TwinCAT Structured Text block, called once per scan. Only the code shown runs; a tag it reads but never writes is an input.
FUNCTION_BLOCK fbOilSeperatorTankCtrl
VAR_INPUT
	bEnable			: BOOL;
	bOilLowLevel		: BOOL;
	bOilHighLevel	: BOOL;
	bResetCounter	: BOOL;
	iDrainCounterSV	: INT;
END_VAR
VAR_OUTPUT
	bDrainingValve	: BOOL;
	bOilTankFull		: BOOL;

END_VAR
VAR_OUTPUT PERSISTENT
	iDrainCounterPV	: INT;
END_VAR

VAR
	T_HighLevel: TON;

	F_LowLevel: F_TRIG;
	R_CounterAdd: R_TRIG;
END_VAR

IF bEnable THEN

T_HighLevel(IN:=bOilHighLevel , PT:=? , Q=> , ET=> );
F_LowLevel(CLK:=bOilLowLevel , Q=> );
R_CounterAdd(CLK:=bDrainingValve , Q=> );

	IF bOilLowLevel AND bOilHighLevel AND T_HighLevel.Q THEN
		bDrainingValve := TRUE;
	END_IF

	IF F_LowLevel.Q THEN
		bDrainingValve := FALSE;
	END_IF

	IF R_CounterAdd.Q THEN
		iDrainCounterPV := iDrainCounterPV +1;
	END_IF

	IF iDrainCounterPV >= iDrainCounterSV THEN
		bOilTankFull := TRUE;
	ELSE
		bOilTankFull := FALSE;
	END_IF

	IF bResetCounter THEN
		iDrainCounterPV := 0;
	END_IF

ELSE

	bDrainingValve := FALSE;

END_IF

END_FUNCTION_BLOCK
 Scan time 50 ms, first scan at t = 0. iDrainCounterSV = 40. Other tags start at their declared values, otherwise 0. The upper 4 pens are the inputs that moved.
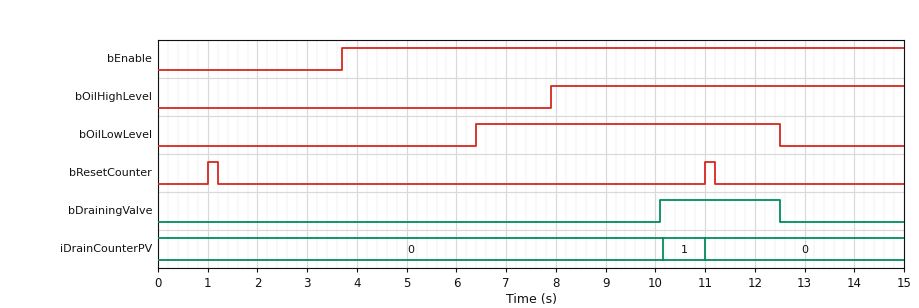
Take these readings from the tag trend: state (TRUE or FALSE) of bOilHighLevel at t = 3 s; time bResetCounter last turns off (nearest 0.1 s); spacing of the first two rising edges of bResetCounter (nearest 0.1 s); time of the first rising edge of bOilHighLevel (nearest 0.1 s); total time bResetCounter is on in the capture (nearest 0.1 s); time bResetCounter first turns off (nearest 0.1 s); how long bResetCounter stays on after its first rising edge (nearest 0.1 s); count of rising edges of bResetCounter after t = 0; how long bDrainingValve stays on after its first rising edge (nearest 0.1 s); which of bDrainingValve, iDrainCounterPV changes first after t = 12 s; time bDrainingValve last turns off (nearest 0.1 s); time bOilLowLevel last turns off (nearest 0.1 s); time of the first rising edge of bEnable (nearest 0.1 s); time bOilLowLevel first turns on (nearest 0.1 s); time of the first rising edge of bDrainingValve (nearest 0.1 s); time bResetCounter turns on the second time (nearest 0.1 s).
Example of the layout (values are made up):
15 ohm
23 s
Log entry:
FALSE
11.2 s
10.0 s
7.9 s
0.4 s
1.2 s
0.2 s
2
2.4 s
bDrainingValve
12.5 s
12.5 s
3.7 s
6.4 s
10.1 s
11.0 s
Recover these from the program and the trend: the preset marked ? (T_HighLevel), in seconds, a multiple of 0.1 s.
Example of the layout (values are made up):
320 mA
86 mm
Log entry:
2.2 s
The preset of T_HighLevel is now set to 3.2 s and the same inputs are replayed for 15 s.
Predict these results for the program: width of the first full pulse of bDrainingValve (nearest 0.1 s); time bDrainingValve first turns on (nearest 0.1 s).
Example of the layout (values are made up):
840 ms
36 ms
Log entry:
1.4 s
11.1 s
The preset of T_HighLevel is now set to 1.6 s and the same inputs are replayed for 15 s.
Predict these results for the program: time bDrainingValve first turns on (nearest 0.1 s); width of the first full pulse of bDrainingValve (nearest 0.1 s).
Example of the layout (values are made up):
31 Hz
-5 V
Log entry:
9.5 s
3.0 s
